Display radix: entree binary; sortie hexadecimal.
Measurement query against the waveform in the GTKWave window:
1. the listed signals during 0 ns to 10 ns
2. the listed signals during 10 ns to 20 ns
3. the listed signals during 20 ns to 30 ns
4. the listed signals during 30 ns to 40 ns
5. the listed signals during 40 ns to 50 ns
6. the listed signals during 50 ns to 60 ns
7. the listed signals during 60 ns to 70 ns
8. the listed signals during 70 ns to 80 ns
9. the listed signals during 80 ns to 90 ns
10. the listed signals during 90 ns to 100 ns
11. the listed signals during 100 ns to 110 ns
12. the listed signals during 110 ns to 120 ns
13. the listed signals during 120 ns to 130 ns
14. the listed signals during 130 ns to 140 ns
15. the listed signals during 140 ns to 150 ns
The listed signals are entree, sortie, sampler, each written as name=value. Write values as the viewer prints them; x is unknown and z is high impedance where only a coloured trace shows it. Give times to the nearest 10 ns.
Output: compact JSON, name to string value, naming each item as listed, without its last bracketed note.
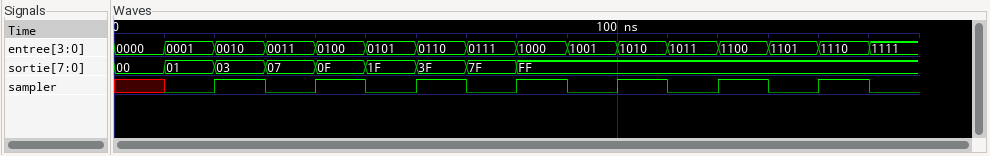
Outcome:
{"the listed signals during 0 ns to 10 ns": "entree=0000, sortie=00, sampler=x", "the listed signals during 10 ns to 20 ns": "entree=0001, sortie=01, sampler=0", "the listed signals during 20 ns to 30 ns": "entree=0010, sortie=03, sampler=1", "the listed signals during 30 ns to 40 ns": "entree=0011, sortie=07, sampler=0", "the listed signals during 40 ns to 50 ns": "entree=0100, sortie=0F, sampler=1", "the listed signals during 50 ns to 60 ns": "entree=0101, sortie=1F, sampler=0", "the listed signals during 60 ns to 70 ns": "entree=0110, sortie=3F, sampler=1", "the listed signals during 70 ns to 80 ns": "entree=0111, sortie=7F, sampler=0", "the listed signals during 80 ns to 90 ns": "entree=1000, sortie=FF, sampler=1", "the listed signals during 90 ns to 100 ns": "entree=1001, sortie=FF, sampler=0", "the listed signals during 100 ns to 110 ns": "entree=1010, sortie=FF, sampler=1", "the listed signals during 110 ns to 120 ns": "entree=1011, sortie=FF, sampler=0", "the listed signals during 120 ns to 130 ns": "entree=1100, sortie=FF, sampler=1", "the listed signals during 130 ns to 140 ns": "entree=1101, sortie=FF, sampler=0", "the listed signals during 140 ns to 150 ns": "entree=1110, sortie=FF, sampler=1"}
